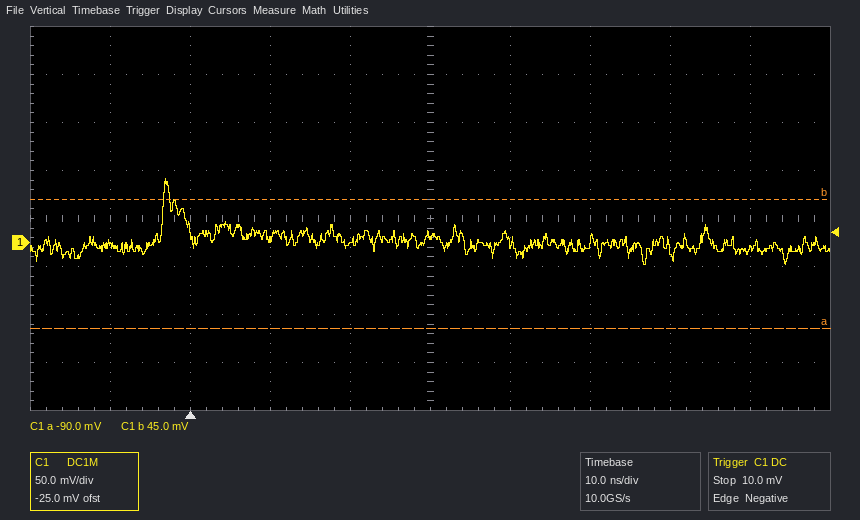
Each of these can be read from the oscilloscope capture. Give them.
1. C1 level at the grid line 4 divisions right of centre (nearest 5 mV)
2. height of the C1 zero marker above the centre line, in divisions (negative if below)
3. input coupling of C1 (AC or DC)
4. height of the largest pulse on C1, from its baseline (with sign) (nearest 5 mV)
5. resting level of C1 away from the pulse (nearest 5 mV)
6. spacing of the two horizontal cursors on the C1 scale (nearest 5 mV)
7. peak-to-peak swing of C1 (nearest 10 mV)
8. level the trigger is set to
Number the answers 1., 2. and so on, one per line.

1. -10 mV
2. -0.5 div
3. DC
4. +70 mV
5. 0 mV
6. 135 mV
7. 90 mV
8. 10.0 mV
